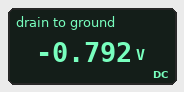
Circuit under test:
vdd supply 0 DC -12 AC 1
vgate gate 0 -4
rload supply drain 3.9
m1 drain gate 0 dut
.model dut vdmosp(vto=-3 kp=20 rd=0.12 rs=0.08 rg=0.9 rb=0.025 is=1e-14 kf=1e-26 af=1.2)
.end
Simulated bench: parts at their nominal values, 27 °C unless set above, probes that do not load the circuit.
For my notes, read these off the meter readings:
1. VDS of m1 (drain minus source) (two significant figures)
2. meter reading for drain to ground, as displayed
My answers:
-790 mV
-0.792 V
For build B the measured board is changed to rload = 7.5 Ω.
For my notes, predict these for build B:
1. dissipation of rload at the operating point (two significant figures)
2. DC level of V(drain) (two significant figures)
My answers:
18 W
-400 mV
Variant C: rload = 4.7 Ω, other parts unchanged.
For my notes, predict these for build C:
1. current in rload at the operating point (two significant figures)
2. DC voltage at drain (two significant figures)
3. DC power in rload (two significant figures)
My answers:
2.4 A
-650 mV
27 W
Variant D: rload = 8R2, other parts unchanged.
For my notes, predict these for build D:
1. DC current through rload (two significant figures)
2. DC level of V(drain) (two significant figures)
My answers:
1.4 A
-370 mV
